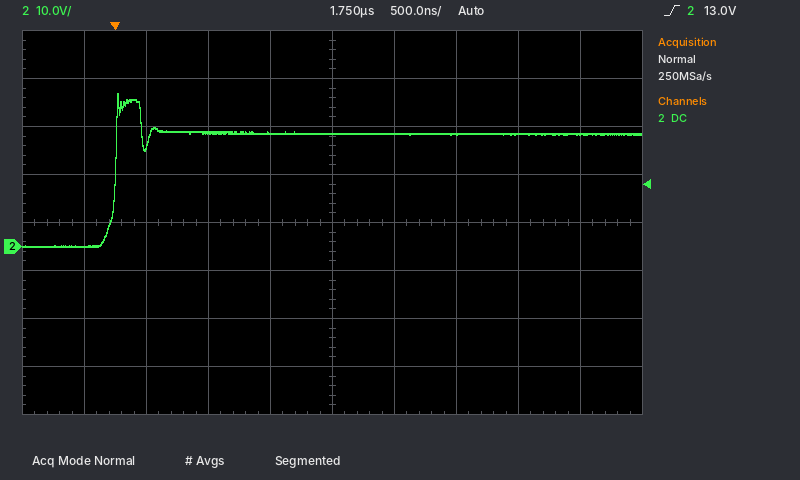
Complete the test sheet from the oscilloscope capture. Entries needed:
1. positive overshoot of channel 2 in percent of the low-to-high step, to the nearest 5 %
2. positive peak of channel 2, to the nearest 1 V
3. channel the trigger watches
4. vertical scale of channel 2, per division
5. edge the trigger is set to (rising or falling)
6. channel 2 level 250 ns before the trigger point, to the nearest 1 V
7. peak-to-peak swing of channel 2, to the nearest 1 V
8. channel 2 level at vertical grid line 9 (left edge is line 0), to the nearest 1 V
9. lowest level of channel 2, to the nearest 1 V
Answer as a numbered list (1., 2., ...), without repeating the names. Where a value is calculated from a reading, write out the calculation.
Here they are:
1. 35 %
2. 32 V
3. channel 2
4. 10 V
5. rising
6. 0 V
7. 32 V − (0 V) = 32 V
8. 23 V
9. 0 V
